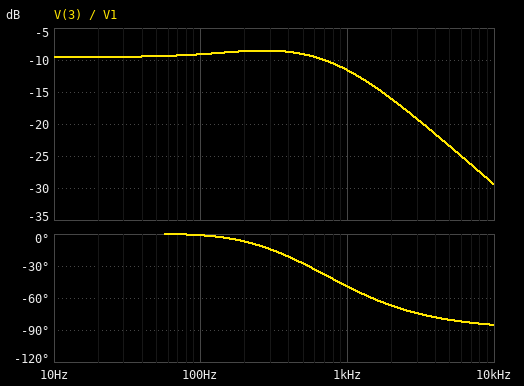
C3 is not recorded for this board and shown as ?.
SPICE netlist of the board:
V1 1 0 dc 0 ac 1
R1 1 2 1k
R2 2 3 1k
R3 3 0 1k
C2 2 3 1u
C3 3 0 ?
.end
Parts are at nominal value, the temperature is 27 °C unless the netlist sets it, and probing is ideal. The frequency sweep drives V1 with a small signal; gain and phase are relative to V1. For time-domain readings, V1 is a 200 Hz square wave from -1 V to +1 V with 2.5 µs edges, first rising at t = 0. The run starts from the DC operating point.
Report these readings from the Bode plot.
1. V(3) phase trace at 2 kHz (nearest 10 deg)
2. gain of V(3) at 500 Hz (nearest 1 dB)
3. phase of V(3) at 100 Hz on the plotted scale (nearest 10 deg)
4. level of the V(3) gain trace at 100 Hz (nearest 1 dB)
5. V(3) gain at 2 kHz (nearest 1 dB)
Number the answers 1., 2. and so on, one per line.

1. -70 deg
2. -9 dB
3. 0 deg
4. -9 dB
5. -16 dB
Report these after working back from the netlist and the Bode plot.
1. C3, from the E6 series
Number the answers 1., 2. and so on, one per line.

1. 470 nF
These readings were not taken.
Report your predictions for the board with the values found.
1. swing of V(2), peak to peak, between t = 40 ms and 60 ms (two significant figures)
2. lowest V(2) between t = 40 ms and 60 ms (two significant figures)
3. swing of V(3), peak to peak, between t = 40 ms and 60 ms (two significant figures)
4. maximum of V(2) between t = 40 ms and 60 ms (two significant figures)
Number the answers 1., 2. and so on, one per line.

1. 1.3 V
2. -660 mV
3. 810 mV
4. 660 mV
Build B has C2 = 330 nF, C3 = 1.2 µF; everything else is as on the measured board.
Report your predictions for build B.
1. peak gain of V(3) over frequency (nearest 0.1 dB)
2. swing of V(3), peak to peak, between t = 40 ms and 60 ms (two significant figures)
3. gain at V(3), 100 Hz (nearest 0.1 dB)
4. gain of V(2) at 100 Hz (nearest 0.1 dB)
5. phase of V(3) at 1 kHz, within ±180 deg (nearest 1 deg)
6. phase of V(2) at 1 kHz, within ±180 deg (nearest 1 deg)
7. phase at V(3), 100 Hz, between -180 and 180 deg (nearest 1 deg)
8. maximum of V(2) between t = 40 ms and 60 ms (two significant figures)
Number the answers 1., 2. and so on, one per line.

1. -9.5 dB
2. 610 mV
3. -10.5 dB
4. -3.8 dB
5. -59 deg
6. -45 deg
7. -22 deg
8. 660 mV
